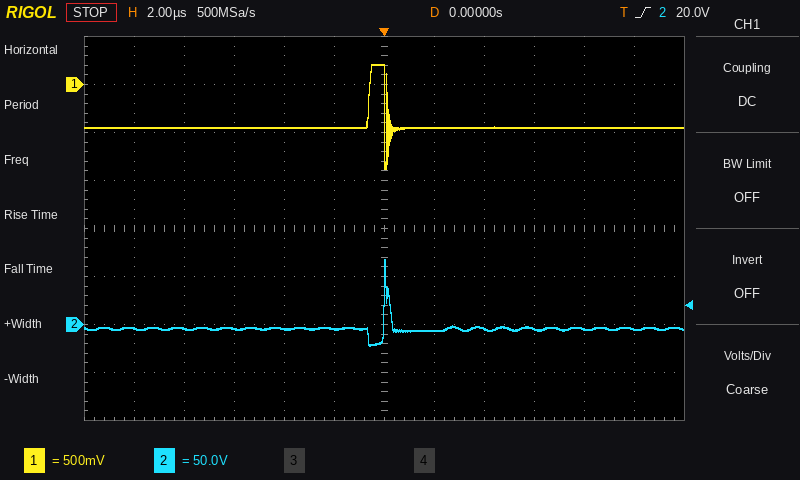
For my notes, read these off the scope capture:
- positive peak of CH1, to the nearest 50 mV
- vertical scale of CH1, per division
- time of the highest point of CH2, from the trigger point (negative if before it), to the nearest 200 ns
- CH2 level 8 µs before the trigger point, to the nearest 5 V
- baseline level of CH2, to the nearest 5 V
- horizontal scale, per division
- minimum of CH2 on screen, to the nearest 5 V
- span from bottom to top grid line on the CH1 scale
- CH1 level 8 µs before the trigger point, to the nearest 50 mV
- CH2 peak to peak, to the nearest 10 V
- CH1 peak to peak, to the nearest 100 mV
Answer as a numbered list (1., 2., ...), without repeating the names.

1. 200 mV
2. 500 mV
3. 0.0 µs
4. -5 V
5. -5 V
6. 2 µs
7. -20 V
8. 4 V
9. -450 mV
10. 90 V
11. 1.10 V
